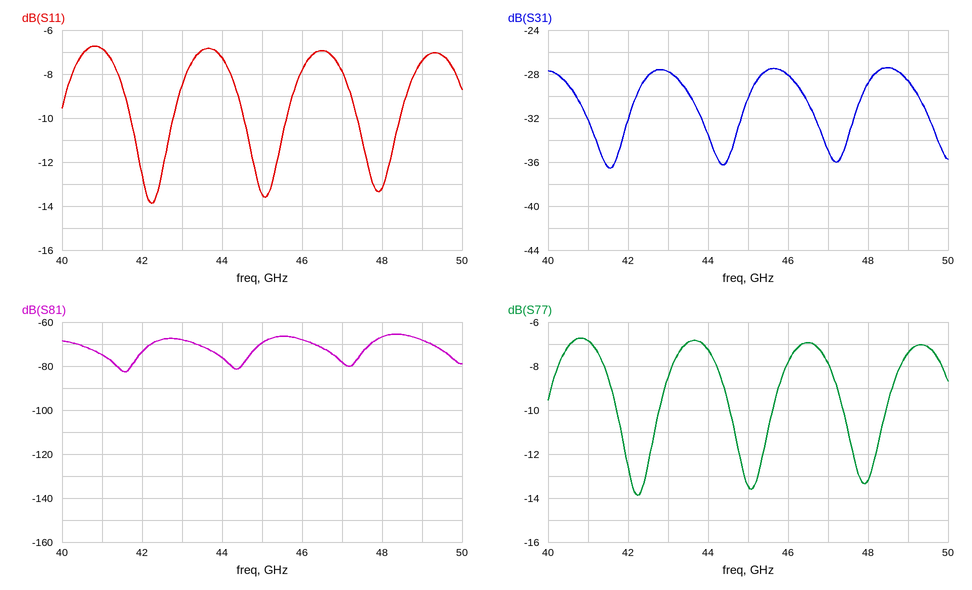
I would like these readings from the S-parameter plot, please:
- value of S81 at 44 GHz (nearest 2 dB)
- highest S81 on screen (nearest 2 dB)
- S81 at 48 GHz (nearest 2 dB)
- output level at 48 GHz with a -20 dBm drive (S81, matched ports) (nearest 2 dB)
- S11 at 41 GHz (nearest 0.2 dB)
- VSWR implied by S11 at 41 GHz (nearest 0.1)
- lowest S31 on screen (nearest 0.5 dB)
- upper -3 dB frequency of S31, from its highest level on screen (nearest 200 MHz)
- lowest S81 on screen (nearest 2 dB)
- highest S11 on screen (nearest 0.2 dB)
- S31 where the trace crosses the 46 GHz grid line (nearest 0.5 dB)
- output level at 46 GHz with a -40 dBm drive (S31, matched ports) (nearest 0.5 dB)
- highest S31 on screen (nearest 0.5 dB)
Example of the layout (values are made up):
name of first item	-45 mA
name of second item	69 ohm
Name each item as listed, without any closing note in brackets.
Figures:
value of S81 at 44 GHz	-76 dB
highest S81 on screen	-66 dB
S81 at 48 GHz	-66 dB
output level at 48 GHz with a -20 dBm drive (S81, matched ports)	-86 dBm
S11 at 41 GHz	-6.8 dB
VSWR implied by S11 at 41 GHz	2.7
lowest S31 on screen	-36.5 dB
upper -3 dB frequency of S31, from its highest level on screen	49.4 GHz
lowest S81 on screen	-82 dB
highest S11 on screen	-6.8 dB
S31 where the trace crosses the 46 GHz grid line	-28.0 dB
output level at 46 GHz with a -40 dBm drive (S31, matched ports)	-68.0 dBm
highest S31 on screen	-27.5 dB
